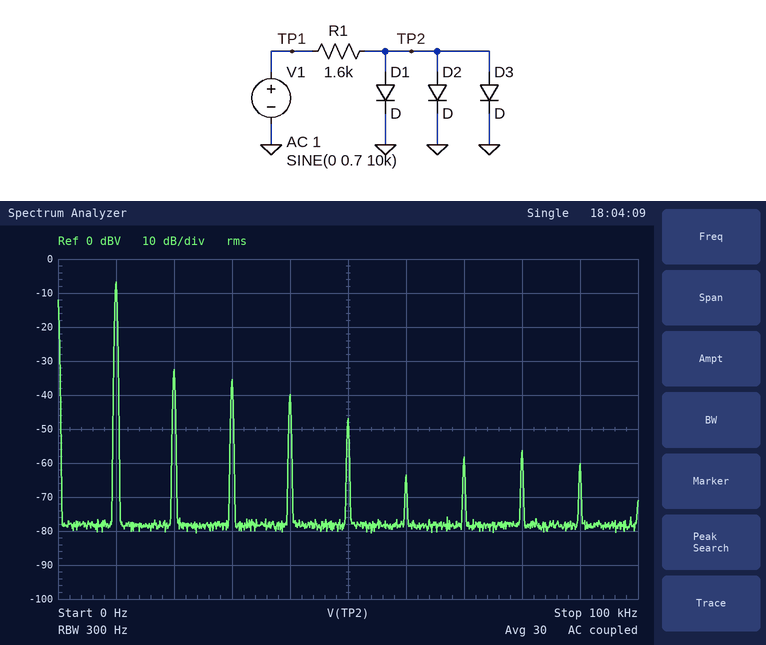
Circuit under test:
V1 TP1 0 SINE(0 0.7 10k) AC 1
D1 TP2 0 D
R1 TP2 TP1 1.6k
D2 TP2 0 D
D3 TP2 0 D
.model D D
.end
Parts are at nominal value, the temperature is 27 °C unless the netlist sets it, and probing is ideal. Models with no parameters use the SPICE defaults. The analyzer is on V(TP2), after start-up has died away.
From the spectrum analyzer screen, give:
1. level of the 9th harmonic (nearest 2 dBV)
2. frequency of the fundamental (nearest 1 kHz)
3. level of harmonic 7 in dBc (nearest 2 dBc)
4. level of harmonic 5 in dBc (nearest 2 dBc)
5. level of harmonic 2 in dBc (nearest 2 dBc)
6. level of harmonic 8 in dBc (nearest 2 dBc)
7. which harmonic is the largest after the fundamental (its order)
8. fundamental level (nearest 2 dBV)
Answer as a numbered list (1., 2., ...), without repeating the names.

1. -60 dBV
2. 10 kHz
3. -52 dBc
4. -40 dBc
5. -26 dBc
6. -50 dBc
7. 2
8. -6 dBV
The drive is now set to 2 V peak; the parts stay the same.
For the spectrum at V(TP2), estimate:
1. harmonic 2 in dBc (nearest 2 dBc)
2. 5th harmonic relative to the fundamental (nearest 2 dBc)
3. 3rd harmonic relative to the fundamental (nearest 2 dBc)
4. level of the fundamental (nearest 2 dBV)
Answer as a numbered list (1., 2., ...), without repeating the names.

1. -12 dBc
2. -30 dBc
3. -22 dBc
4. 0 dBV
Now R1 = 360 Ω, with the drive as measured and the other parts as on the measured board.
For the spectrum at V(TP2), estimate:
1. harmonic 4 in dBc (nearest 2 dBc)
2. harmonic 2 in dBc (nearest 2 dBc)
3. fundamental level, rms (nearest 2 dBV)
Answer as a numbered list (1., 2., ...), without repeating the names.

1. -34 dBc
2. -28 dBc
3. -6 dBV
